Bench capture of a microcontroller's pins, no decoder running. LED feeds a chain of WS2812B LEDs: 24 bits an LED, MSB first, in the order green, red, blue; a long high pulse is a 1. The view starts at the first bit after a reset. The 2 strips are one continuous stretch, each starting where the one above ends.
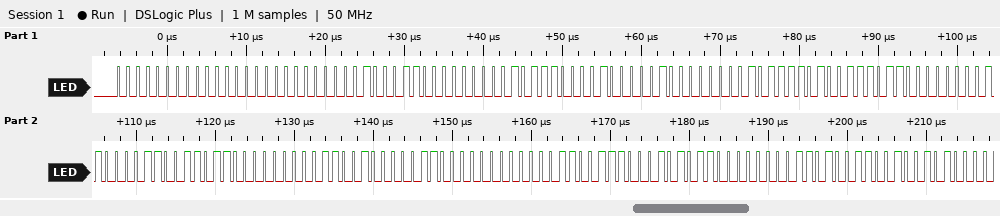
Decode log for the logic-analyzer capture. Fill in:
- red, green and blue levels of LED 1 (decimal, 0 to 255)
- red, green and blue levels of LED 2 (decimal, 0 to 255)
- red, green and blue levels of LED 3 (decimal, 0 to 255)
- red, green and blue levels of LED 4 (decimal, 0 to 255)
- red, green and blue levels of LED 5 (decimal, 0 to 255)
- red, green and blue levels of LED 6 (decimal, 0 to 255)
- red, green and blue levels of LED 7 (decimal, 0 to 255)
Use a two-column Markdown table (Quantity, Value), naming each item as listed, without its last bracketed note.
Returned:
| Quantity | Value |
|---|---|
| red, green and blue levels of LED 1 | 0, 0, 0 |
| red, green and blue levels of LED 2 | 0, 70, 184 |
| red, green and blue levels of LED 3 | 0, 65, 189 |
| red, green and blue levels of LED 4 | 0, 59, 195 |
| red, green and blue levels of LED 5 | 0, 54, 200 |
| red, green and blue levels of LED 6 | 0, 48, 206 |
| red, green and blue levels of LED 7 | 0, 43, 211 |
